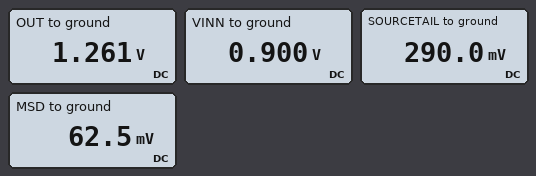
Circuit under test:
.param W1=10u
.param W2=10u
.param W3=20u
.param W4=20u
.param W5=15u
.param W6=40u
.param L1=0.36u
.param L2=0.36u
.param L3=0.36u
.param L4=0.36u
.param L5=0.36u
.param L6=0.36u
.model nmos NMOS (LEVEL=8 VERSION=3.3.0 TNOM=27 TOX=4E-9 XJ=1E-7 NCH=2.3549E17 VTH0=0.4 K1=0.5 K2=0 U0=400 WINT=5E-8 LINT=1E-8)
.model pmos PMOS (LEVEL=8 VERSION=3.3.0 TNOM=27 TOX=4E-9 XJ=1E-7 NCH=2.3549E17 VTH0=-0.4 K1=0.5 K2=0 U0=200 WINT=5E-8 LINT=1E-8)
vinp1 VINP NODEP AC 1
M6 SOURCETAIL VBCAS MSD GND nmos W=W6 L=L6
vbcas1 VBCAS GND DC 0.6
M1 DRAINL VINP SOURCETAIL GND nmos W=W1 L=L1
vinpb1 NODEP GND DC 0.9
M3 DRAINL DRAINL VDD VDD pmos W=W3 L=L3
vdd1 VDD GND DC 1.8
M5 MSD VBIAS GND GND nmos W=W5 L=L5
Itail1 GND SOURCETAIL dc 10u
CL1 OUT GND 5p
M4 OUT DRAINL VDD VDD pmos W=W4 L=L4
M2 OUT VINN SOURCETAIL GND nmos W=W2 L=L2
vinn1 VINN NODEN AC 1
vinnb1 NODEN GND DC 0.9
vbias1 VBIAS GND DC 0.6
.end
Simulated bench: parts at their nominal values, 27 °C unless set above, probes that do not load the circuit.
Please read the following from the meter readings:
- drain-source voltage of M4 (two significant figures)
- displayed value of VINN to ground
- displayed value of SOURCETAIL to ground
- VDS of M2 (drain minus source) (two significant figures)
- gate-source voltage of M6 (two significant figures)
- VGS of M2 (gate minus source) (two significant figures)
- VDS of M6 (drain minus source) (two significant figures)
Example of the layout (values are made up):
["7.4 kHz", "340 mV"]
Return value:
["-540 mV", "0.900 V", "290.0 mV", "970 mV", "540 mV", "610 mV", "230 mV"]
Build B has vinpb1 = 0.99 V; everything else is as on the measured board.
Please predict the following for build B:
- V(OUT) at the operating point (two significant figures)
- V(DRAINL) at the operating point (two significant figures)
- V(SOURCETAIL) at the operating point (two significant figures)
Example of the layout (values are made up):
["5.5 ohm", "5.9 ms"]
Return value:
["1.8 V", "1.2 V", "340 mV"]
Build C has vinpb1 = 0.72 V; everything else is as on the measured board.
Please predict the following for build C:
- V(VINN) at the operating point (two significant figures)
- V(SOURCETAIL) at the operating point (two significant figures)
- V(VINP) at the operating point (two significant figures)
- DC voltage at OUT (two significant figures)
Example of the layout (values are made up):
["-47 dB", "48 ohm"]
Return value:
["900 mV", "150 mV", "720 mV", "160 mV"]
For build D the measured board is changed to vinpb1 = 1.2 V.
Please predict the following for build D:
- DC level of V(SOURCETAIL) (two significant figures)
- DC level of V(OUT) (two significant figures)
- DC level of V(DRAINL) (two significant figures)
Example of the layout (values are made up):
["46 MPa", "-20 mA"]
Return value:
["510 mV", "1.8 V", "1.2 V"]
